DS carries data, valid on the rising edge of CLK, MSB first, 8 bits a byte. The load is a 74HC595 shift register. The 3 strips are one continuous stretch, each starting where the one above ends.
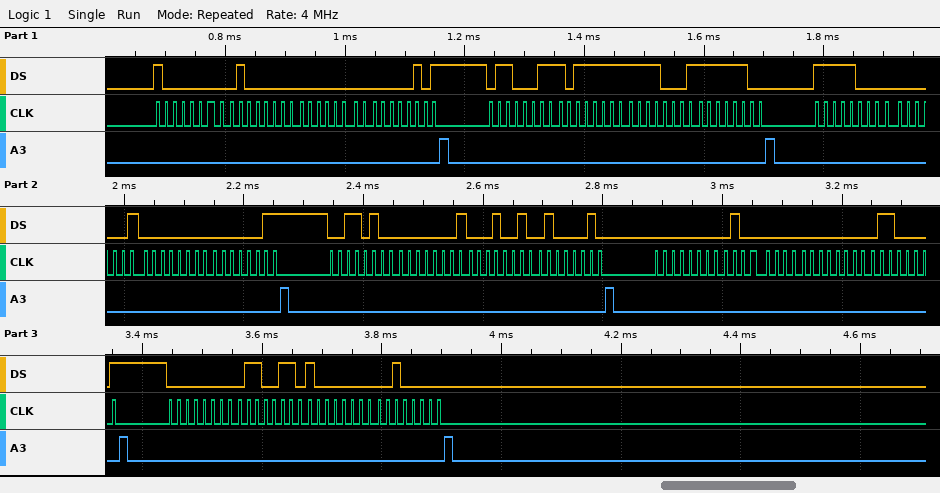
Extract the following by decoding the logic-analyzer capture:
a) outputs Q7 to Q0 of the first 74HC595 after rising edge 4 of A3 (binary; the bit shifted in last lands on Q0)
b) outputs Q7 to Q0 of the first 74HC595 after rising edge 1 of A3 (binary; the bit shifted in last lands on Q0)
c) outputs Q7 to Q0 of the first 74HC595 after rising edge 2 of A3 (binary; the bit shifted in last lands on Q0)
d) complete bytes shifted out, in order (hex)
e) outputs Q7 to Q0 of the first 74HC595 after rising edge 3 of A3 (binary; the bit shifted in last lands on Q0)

01000010
00000101
11111100
80 40 00 05 63 BF F1 FC F8 01 00 03 34 01 12 42 00 40 00 61 00 66 80 20
00000011
